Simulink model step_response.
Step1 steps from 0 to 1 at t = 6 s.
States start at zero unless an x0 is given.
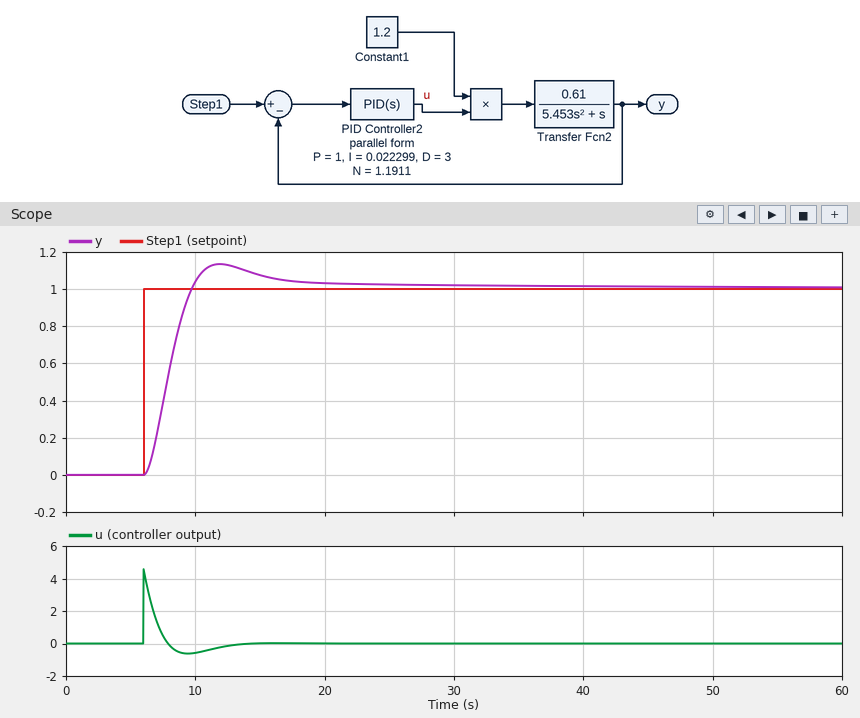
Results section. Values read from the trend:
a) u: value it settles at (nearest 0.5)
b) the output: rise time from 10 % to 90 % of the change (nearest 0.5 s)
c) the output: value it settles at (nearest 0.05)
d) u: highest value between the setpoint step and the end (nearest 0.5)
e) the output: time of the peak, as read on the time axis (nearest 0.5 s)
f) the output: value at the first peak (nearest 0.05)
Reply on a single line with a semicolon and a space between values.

0.0; 2.5 s; 1.00; 4.5; 12.0 s; 1.15
